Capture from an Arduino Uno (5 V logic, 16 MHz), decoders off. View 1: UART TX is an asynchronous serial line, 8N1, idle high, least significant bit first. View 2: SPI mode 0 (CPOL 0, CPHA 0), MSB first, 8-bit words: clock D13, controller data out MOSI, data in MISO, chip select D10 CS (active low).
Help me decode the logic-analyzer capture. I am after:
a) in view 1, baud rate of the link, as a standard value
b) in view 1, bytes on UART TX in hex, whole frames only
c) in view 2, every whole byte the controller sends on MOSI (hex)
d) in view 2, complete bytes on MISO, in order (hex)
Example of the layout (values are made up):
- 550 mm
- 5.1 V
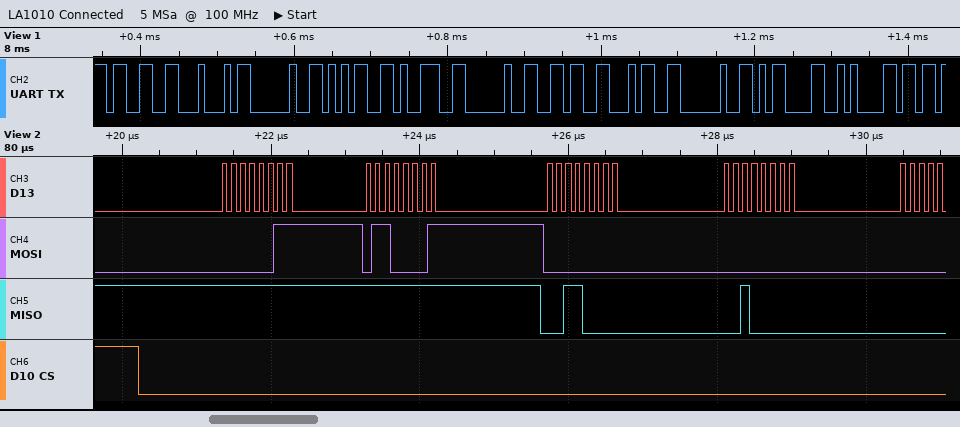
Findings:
- 115200 baud
- 33 44 20 35 39 20 36 34 20 0D 0A
- 0x03 0x61 0x00 0x00
- 0xFF 0xFF 0x30 0x20
